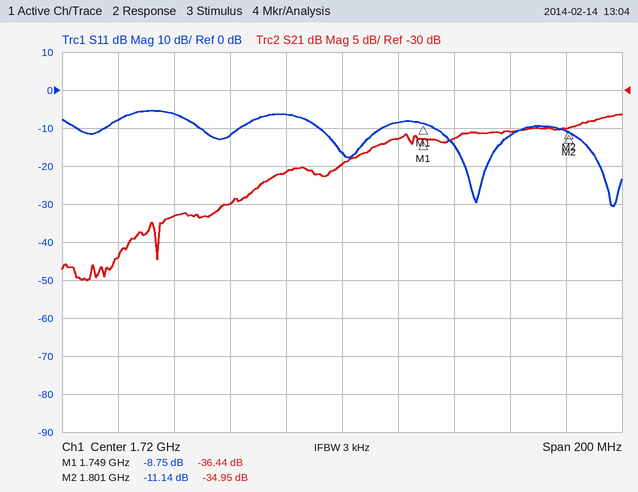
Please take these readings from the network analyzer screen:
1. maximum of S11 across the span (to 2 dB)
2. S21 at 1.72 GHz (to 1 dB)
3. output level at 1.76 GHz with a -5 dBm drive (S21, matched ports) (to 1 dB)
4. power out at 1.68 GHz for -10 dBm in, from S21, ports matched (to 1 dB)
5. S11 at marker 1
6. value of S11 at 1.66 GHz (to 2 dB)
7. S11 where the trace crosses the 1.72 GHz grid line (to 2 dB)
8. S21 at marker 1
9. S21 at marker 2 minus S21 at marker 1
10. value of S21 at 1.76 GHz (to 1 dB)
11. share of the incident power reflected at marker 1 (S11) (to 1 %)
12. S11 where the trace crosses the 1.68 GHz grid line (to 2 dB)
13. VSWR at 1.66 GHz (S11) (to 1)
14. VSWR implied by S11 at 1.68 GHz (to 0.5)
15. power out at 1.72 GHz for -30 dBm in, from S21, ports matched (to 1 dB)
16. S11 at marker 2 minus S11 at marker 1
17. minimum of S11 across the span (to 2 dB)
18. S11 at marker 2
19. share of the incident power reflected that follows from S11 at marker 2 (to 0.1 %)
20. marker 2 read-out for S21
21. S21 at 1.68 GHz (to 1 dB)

-6 dB
-40 dB
-41 dBm
-55 dBm
-8.75 dB
-6 dB
-16 dB
-36.44 dB
1.49 dB
-36 dB
13 %
-12 dB
3
1.5
-70 dBm
-2.39 dB
-30 dB
-11.14 dB
7.7 %
-34.95 dB
-45 dB
